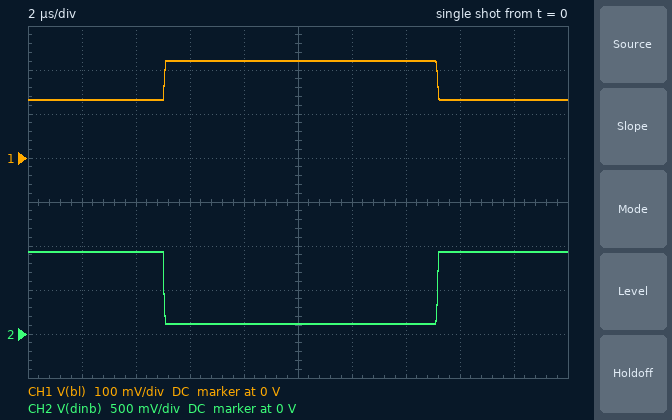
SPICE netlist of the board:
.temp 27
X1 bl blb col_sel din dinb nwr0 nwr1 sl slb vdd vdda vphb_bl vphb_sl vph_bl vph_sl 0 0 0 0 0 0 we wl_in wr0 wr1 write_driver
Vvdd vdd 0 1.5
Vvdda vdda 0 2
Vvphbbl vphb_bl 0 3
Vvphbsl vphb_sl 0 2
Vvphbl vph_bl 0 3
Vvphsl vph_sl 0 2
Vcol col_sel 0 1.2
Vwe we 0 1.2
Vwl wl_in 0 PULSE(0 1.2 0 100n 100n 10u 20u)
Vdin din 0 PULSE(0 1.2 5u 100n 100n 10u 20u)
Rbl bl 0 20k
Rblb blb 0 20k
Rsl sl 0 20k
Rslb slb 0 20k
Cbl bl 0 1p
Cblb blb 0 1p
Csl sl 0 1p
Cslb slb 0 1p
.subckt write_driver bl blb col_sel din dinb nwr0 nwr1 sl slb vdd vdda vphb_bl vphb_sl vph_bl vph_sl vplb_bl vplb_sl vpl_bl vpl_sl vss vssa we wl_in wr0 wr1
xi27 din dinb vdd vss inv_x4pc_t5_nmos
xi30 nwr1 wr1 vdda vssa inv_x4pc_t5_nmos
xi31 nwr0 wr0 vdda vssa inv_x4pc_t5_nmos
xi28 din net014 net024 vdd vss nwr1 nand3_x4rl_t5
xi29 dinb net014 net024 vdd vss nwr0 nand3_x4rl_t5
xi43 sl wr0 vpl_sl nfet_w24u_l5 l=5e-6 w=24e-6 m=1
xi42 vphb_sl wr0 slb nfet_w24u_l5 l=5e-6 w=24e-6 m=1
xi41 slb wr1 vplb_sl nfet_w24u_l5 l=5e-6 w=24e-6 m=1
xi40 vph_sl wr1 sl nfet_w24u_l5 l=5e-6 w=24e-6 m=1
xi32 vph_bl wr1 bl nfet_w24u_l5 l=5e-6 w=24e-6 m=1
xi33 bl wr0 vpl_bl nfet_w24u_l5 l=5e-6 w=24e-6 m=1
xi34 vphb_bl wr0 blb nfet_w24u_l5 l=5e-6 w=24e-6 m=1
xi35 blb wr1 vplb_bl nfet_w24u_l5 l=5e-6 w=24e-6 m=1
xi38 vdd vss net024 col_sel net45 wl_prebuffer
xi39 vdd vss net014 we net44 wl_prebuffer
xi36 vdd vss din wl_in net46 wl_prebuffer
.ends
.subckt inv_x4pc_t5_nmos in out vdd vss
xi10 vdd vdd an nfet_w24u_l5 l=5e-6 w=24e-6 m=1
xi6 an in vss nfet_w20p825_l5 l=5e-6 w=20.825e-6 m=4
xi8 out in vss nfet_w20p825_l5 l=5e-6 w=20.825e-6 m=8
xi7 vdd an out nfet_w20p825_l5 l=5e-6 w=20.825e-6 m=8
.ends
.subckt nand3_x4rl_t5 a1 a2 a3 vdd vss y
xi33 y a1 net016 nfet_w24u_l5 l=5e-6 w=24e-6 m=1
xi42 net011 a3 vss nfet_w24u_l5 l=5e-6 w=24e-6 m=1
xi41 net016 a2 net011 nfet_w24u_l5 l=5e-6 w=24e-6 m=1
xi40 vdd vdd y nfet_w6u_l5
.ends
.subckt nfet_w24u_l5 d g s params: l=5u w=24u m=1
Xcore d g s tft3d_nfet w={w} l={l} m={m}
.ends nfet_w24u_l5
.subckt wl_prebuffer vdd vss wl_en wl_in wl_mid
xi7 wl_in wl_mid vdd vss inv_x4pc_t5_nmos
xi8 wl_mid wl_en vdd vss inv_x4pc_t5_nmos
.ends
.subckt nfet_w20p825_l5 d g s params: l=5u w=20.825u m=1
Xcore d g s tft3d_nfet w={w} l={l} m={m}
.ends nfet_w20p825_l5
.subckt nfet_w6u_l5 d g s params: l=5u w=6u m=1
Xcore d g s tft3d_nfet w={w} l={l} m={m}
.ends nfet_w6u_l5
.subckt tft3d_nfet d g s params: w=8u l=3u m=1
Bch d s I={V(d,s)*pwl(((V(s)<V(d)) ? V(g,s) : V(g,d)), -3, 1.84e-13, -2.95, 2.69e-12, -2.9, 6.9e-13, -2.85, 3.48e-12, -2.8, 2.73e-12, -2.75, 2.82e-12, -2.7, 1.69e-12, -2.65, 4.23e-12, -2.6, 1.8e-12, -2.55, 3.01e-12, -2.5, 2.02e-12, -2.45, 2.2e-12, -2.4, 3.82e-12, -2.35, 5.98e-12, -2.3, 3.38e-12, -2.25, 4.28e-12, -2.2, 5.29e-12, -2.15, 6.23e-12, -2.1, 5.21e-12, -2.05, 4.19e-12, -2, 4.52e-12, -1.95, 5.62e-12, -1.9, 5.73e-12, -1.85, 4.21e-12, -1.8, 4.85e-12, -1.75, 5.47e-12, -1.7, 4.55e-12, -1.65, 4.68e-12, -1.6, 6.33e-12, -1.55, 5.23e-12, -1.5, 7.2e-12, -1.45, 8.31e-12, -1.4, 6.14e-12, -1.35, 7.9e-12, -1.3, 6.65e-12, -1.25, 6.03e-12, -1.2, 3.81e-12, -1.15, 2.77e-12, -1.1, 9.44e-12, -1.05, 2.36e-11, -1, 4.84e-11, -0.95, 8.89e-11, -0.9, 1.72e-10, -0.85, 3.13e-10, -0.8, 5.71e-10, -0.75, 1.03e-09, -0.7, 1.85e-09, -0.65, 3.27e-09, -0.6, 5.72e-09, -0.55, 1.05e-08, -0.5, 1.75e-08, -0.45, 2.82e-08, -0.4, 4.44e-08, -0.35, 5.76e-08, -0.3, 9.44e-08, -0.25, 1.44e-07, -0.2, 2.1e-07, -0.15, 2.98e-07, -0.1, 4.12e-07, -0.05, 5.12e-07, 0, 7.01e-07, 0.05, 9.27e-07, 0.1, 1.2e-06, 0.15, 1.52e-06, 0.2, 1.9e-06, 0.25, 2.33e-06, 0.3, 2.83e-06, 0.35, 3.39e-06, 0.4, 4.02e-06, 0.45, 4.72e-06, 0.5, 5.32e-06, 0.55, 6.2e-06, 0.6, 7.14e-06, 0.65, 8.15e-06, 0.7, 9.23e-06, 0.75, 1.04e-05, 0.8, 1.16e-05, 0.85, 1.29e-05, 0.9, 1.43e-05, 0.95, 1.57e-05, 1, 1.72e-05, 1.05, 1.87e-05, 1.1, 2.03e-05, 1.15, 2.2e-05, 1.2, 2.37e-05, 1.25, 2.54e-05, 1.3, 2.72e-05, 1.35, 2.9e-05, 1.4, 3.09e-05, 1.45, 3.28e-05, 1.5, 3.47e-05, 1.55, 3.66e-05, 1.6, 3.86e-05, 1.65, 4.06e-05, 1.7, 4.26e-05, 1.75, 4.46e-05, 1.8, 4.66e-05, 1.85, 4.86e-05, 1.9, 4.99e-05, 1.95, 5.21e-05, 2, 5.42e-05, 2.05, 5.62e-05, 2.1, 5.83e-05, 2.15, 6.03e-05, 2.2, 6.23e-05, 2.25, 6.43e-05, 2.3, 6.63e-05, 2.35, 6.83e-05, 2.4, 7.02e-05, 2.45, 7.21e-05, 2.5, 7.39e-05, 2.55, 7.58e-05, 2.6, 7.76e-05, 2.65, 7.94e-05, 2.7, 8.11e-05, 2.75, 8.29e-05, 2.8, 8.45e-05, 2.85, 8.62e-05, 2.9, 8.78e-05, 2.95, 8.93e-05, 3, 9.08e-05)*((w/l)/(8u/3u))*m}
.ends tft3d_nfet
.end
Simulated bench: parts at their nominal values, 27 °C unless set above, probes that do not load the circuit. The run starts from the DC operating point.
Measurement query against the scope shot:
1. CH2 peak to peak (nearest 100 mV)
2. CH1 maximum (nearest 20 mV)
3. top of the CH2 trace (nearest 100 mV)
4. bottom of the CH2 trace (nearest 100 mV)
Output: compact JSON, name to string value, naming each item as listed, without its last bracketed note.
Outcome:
{"CH2 peak to peak": "800 mV", "CH1 maximum": "220 mV", "top of the CH2 trace": "900 mV", "bottom of the CH2 trace": "100 mV"}
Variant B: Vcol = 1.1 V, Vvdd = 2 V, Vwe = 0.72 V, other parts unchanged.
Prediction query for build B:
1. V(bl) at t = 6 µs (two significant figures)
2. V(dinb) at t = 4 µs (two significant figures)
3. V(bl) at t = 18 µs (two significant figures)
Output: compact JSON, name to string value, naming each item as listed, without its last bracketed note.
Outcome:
{"V(bl) at t = 6 µs": "130 mV", "V(dinb) at t = 4 µs": "1.3 V", "V(bl) at t = 18 µs": "92 mV"}
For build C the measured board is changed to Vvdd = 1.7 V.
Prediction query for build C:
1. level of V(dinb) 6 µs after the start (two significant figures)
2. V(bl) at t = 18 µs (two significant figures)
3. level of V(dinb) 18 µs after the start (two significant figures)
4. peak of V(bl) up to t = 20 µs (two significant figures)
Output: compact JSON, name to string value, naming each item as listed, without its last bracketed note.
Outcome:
{"level of V(dinb) 6 µs after the start": "160 mV", "V(bl) at t = 18 µs": "110 mV", "level of V(dinb) 18 µs after the start": "1.1 V", "peak of V(bl) up to t = 20 µs": "190 mV"}
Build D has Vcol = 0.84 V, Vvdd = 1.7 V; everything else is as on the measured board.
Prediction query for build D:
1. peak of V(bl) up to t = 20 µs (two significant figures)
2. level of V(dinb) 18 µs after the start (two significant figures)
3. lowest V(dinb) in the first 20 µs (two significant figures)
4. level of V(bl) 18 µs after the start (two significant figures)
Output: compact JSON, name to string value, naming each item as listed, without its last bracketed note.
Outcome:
{"peak of V(bl) up to t = 20 µs": "180 mV", "level of V(dinb) 18 µs after the start": "1.1 V", "lowest V(dinb) in the first 20 µs": "160 mV", "level of V(bl) 18 µs after the start": "110 mV"}
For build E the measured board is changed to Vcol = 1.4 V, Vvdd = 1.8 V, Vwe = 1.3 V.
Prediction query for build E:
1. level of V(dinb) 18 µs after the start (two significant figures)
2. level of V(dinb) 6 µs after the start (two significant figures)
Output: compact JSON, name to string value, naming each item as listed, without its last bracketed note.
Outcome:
{"level of V(dinb) 18 µs after the start": "1.2 V", "level of V(dinb) 6 µs after the start": "180 mV"}
